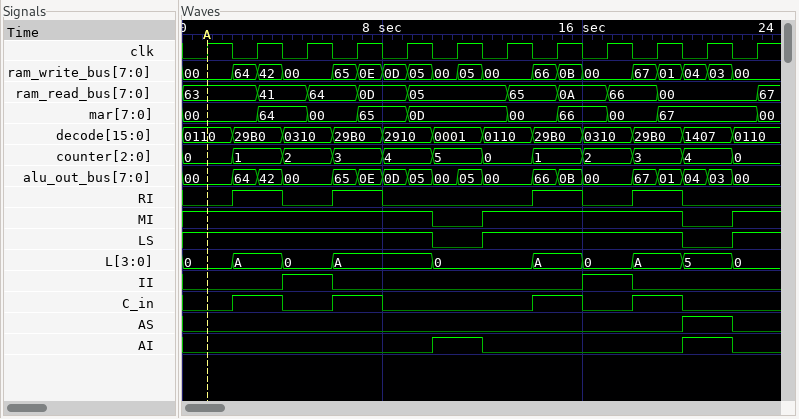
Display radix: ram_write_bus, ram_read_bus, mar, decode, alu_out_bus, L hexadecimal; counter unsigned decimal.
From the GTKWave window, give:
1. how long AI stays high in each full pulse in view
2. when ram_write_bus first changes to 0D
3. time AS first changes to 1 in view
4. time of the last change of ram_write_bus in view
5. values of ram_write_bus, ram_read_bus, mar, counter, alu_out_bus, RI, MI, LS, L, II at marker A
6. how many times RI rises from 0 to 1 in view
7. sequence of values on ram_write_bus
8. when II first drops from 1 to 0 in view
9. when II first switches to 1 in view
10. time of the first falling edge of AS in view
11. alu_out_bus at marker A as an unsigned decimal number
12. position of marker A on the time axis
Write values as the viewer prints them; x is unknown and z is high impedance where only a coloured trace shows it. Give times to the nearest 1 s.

2 s, 2 s
8 s
20 s
22 s
ram_write_bus=00, ram_read_bus=63, mar=00, counter=0, alu_out_bus=00, RI=0, MI=1, LS=1, L=0, II=0
4
00, 64, 42, 00, 65, 0E, 0D, 05, 00, 05, 00, 66, 0B, 00, 67, 01, 04, 03, 00
6 s
4 s
22 s
0
1 s
